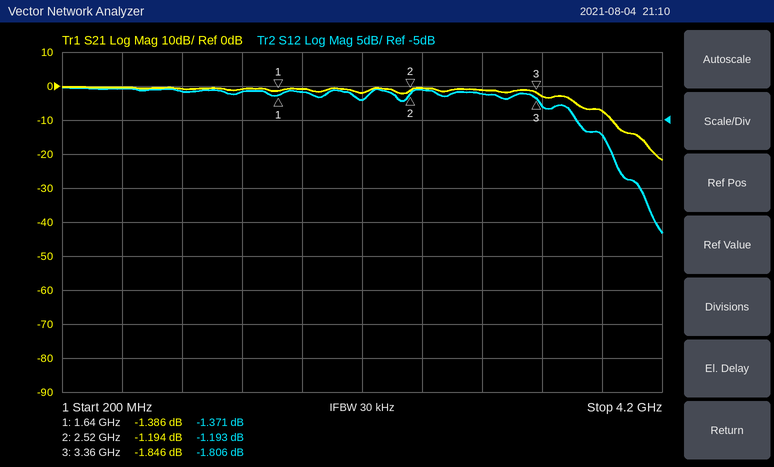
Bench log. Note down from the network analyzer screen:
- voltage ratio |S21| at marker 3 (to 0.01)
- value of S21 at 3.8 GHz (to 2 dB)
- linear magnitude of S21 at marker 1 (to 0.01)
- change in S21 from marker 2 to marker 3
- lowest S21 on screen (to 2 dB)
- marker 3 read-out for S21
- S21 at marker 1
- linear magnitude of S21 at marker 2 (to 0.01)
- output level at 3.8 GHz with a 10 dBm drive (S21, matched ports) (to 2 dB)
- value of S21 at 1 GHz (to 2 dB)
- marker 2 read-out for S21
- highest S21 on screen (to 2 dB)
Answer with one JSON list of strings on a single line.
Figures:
["0.81", "-8 dB", "0.85", "-0.652 dB", "-22 dB", "-1.846 dB", "-1.386 dB", "0.87", "2 dBm", "0 dB", "-1.194 dB", "0 dB"]
